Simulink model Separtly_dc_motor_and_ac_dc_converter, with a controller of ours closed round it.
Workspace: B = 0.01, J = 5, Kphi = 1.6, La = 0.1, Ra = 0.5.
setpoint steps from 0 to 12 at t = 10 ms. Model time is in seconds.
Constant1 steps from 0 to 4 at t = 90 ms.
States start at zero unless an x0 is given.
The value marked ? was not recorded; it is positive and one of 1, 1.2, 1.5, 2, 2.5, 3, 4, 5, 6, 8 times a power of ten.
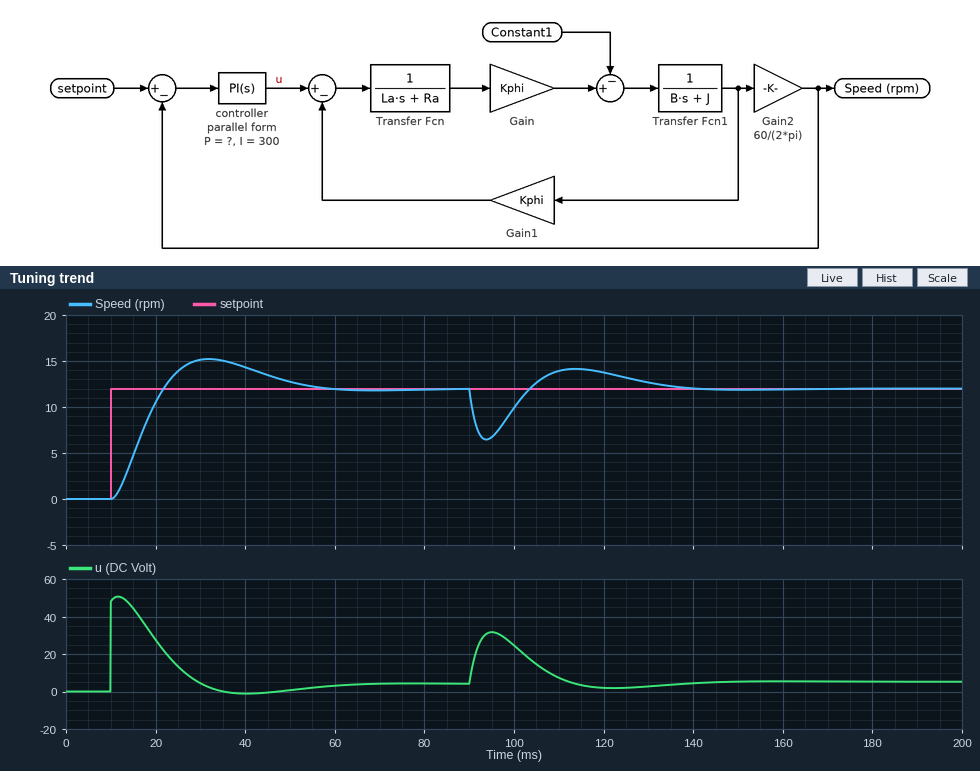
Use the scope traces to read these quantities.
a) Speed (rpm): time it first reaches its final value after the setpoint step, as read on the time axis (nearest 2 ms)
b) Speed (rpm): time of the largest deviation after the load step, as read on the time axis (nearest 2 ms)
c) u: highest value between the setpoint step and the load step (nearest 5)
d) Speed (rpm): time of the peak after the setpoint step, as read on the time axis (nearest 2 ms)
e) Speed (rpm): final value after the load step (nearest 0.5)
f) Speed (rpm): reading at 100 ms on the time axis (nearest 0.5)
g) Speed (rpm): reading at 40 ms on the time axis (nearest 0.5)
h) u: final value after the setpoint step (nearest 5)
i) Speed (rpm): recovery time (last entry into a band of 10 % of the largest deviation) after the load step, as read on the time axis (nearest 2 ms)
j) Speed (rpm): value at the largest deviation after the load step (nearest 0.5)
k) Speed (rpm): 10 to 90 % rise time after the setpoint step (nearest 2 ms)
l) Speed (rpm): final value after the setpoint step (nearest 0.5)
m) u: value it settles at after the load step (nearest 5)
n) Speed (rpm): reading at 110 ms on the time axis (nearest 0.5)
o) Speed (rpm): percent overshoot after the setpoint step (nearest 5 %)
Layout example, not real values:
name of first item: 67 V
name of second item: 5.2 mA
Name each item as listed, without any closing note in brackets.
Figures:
Speed (rpm): time it first reaches its final value after the setpoint step, as read on the time axis: 22 ms
Speed (rpm): time of the largest deviation after the load step, as read on the time axis: 94 ms
u: highest value between the setpoint step and the load step: 50
Speed (rpm): time of the peak after the setpoint step, as read on the time axis: 32 ms
Speed (rpm): final value after the load step: 12.0
Speed (rpm): reading at 100 ms on the time axis: 10.0
Speed (rpm): reading at 40 ms on the time axis: 14.5
u: final value after the setpoint step: 5
Speed (rpm): recovery time (last entry into a band of 10 % of the largest deviation) after the load step, as read on the time axis: 132 ms
Speed (rpm): value at the largest deviation after the load step: 6.5
Speed (rpm): 10 to 90 % rise time after the setpoint step: 8 ms
Speed (rpm): final value after the setpoint step: 12.0
u: value it settles at after the load step: 5
Speed (rpm): reading at 110 ms on the time axis: 14.0
Speed (rpm): percent overshoot after the setpoint step: 25 %
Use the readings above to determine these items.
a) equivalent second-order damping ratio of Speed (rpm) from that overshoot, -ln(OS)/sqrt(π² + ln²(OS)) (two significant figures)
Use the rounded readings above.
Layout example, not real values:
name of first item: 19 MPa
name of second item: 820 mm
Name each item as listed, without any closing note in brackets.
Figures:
equivalent second-order damping ratio of Speed (rpm) from that overshoot, -ln(OS)/sqrt(π² + ln²(OS)): 0.40
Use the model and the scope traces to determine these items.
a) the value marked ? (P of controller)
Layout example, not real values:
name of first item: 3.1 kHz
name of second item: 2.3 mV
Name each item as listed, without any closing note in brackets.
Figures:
the value marked ?: 4
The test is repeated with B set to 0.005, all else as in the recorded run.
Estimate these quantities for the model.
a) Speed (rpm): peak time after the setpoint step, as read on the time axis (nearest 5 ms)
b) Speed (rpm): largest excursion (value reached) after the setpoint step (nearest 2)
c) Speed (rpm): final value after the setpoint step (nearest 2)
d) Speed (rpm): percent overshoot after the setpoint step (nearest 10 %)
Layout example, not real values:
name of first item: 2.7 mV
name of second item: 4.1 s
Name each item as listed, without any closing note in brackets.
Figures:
Speed (rpm): peak time after the setpoint step, as read on the time axis: 35 ms
Speed (rpm): largest excursion (value reached) after the setpoint step: 14
Speed (rpm): final value after the setpoint step: 12
Speed (rpm): percent overshoot after the setpoint step: 20 %
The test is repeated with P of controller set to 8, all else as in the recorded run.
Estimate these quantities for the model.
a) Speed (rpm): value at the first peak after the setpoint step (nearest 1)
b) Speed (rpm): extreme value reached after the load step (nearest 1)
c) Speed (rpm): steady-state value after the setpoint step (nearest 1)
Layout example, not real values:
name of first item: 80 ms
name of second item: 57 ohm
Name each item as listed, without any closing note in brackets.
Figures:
Speed (rpm): value at the first peak after the setpoint step: 14
Speed (rpm): extreme value reached after the load step: 7
Speed (rpm): steady-state value after the setpoint step: 12
